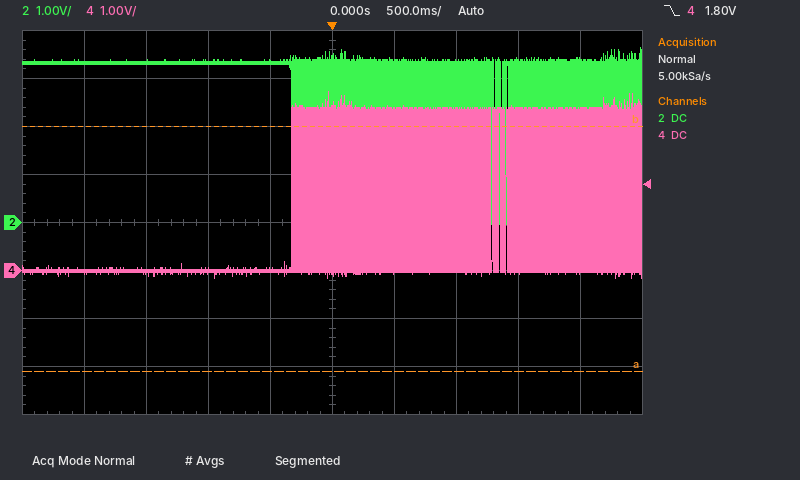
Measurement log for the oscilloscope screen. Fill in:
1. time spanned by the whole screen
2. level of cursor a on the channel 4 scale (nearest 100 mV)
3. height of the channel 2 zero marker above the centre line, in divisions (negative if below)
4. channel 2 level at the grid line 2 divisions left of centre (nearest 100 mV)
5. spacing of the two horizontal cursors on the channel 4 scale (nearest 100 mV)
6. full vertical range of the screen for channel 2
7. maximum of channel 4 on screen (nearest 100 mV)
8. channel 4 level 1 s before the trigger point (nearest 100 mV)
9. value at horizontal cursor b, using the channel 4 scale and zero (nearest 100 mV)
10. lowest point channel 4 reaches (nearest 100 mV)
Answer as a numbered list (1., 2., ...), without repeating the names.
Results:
1. 5 s
2. -2.1 V
3. 0.0 div
4. 3.4 V
5. 5.1 V
6. 8 V
7. 3.7 V
8. 0.0 V
9. 3.0 V
10. -100 mV
